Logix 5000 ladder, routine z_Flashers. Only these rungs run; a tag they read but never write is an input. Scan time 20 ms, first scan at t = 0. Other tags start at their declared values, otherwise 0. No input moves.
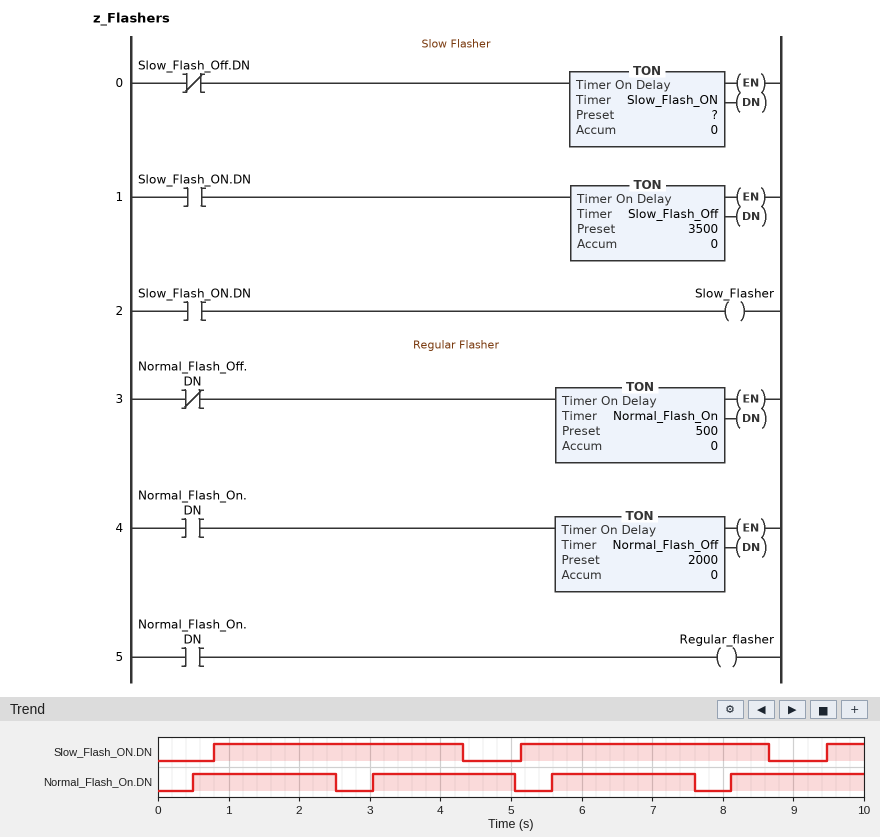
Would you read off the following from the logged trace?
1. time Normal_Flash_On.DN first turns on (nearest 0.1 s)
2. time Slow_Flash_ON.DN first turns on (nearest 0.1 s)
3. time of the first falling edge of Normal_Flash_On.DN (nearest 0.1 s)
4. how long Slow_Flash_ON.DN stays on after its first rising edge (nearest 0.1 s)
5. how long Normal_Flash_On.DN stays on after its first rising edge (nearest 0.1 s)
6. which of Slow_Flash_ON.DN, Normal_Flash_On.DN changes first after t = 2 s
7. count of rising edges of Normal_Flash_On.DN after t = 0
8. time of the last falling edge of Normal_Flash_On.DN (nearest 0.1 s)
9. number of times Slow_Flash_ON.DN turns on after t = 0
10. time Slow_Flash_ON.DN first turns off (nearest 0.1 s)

0.5 s
0.8 s
2.5 s
3.5 s
2.0 s
Normal_Flash_On.DN
4
7.6 s
3
4.3 s
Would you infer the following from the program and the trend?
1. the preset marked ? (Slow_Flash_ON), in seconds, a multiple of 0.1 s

0.8 s
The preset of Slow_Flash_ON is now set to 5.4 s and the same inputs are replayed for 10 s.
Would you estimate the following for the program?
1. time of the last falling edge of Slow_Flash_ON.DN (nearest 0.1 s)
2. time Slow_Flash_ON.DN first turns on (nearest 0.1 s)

8.9 s
5.4 s
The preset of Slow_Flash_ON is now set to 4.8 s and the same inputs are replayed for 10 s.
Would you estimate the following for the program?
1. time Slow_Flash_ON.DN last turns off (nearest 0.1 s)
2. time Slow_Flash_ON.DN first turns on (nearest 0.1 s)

8.3 s
4.8 s
